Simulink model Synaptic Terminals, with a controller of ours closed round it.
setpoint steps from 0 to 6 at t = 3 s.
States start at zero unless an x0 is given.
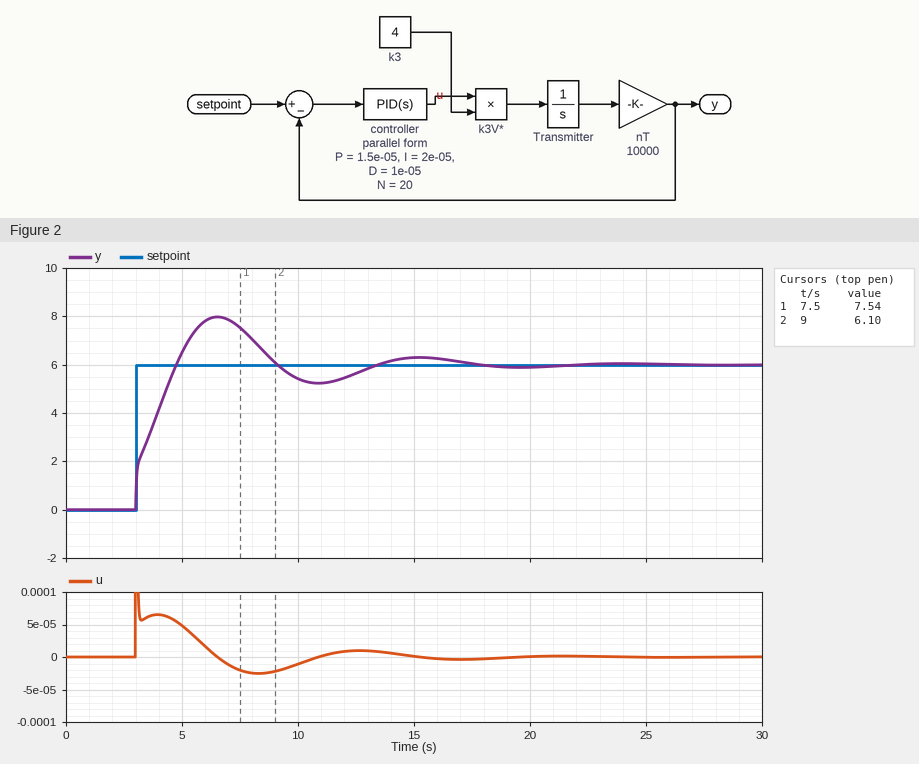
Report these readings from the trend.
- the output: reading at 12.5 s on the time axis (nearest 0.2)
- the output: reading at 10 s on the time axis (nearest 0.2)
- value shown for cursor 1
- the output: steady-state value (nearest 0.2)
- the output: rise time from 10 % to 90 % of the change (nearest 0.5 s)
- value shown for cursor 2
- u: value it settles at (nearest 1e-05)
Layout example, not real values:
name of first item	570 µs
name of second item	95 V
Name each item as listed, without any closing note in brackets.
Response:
the output: reading at 12.5 s on the time axis	5.6
the output: reading at 10 s on the time axis	5.4
value shown for cursor 1	7.54
the output: steady-state value	6.0
the output: rise time from 10 % to 90 % of the change	1.5 s
value shown for cursor 2	6.10
u: value it settles at	0.00000
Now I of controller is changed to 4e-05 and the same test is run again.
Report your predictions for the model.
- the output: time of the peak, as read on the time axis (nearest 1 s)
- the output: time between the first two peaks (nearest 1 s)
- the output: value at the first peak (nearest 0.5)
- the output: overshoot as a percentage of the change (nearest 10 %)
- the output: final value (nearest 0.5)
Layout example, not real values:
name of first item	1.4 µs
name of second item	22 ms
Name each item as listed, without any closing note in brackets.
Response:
the output: time of the peak, as read on the time axis	6 s
the output: time between the first two peaks	6 s
the output: value at the first peak	8.5
the output: overshoot as a percentage of the change	40 %
the output: final value	6.0
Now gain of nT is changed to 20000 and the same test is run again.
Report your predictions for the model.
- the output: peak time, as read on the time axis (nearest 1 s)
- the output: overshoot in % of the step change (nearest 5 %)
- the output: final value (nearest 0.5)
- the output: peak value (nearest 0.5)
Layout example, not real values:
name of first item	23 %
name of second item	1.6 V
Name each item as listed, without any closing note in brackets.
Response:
the output: peak time, as read on the time axis	6 s
the output: overshoot in % of the step change	20 %
the output: final value	6.0
the output: peak value	7.5
